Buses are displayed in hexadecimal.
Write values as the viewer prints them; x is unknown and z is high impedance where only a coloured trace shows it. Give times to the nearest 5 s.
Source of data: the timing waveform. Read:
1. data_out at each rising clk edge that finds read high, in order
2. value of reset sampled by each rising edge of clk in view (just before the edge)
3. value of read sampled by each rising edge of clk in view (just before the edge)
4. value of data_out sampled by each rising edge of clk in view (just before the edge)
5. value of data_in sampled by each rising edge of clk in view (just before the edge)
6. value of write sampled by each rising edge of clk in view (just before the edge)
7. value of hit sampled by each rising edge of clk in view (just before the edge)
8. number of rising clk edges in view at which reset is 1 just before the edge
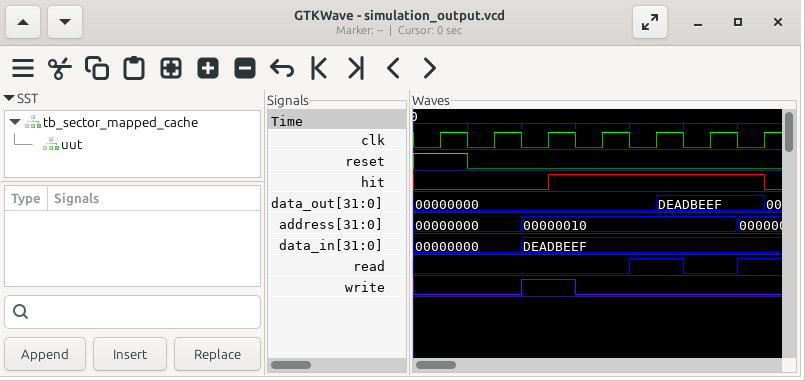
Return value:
00000000, DEADBEEF
1 0 0 0 0 0 0
0 0 0 0 1 0 1
00000000, 00000000, 00000000, 00000000, 00000000, DEADBEEF, DEADBEEF
00000000, 00000000, DEADBEEF, DEADBEEF, DEADBEEF, DEADBEEF, DEADBEEF
0 0 1 0 0 0 0
0 0 0 1 1 1 1
1
